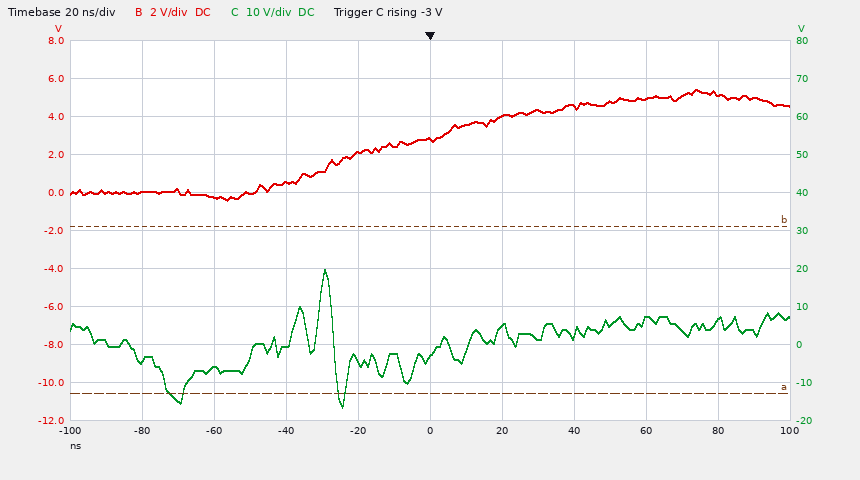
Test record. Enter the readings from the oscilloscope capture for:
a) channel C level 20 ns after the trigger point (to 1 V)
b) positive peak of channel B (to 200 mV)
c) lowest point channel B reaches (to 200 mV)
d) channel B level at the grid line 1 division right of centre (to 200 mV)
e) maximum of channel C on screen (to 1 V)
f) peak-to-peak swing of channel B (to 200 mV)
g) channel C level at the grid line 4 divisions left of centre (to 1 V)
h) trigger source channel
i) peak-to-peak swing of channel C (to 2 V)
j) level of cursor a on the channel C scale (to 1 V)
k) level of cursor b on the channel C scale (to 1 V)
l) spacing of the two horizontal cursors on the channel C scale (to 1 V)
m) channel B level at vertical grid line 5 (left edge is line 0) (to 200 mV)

5 V
5.4 V
-400 mV
4.0 V
20 V
5.8 V
-4 V
channel C
36 V
-13 V
31 V
44 V
2.8 V
